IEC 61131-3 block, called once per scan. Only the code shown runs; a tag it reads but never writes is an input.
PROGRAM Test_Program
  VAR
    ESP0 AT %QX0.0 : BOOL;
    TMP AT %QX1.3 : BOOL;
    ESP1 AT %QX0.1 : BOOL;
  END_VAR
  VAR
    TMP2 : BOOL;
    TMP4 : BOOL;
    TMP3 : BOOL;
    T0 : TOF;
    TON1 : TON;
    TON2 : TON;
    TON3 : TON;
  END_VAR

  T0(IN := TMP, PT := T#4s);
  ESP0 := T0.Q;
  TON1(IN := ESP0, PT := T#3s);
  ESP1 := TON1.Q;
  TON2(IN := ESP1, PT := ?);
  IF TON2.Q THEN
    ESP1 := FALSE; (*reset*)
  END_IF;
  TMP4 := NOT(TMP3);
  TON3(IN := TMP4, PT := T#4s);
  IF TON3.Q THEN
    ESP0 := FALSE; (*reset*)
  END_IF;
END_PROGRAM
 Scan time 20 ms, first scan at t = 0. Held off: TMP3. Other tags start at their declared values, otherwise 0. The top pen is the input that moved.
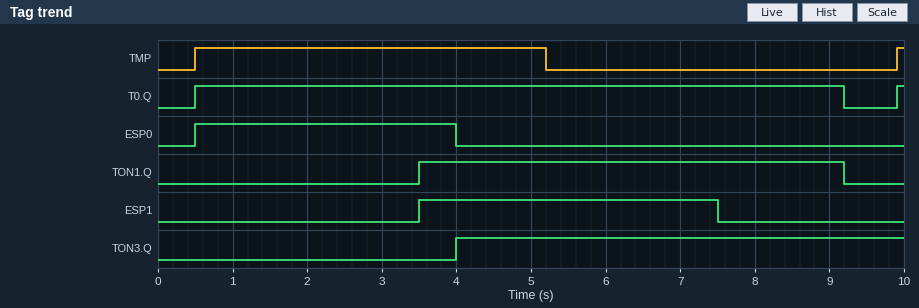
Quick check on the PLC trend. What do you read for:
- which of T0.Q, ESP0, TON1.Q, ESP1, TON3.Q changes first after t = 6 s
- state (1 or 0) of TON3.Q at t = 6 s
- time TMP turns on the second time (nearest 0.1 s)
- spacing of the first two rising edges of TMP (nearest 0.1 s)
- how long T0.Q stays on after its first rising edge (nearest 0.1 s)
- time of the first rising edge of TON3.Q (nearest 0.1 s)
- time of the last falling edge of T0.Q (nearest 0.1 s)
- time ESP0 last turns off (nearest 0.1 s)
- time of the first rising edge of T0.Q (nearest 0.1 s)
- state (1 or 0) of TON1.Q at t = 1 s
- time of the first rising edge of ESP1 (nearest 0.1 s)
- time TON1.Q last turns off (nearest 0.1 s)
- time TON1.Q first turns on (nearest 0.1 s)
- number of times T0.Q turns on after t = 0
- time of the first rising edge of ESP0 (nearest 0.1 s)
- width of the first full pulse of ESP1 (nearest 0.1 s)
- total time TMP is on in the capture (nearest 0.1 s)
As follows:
ESP1
1
9.9 s
9.4 s
8.7 s
4.0 s
9.2 s
4.0 s
0.5 s
0
3.5 s
9.2 s
3.5 s
2
0.5 s
4.0 s
4.8 s
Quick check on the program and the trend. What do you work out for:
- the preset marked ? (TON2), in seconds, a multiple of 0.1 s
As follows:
4.0 s
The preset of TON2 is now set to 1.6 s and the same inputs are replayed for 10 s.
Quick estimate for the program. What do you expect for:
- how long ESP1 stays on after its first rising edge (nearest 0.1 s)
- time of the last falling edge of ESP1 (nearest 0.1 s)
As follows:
1.6 s
5.1 s
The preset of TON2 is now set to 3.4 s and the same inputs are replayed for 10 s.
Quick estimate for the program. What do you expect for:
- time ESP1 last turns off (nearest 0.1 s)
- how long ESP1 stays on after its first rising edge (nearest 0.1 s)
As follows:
6.9 s
3.4 s
